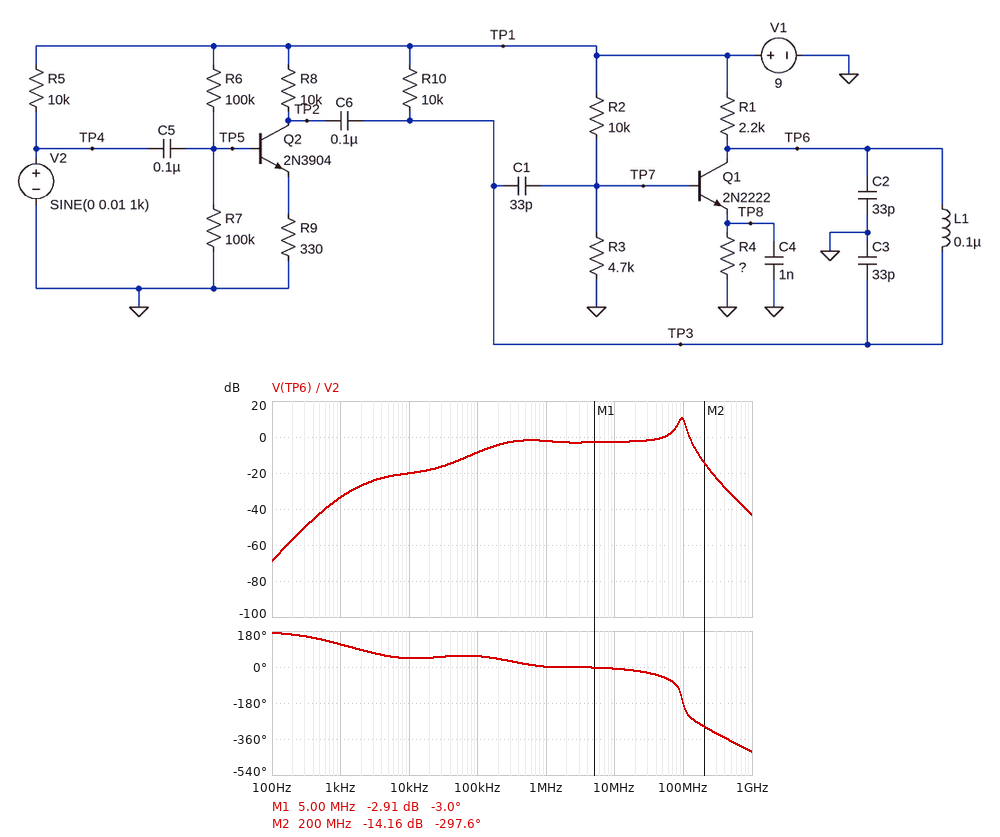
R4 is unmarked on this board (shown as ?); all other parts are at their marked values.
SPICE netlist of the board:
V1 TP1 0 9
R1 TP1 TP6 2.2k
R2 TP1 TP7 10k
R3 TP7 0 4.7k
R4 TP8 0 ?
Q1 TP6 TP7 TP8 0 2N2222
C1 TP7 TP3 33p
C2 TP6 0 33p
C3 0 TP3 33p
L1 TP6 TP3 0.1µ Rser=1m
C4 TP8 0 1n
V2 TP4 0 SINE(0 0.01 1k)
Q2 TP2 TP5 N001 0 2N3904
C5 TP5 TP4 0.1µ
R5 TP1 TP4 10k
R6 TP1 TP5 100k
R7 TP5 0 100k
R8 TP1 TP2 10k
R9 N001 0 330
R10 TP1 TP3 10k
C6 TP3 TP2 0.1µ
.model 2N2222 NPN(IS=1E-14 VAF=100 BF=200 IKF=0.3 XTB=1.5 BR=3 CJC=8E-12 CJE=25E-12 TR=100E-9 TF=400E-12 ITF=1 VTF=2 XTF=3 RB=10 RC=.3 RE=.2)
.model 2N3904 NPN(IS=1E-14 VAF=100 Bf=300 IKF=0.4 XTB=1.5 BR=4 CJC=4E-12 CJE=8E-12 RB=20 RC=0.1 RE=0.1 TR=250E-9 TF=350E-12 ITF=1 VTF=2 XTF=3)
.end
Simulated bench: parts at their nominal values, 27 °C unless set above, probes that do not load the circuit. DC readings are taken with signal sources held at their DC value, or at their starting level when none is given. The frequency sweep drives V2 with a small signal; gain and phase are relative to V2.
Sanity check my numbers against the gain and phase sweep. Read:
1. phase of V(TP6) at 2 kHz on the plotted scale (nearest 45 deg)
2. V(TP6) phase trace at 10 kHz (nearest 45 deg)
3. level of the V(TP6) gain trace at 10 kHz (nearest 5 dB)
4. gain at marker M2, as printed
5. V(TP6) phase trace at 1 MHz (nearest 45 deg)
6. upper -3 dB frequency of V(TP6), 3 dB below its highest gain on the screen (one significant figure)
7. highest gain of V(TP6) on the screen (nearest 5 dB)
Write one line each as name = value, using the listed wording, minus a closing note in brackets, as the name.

phase of V(TP6) at 2 kHz on the plotted scale = 90 deg
V(TP6) phase trace at 10 kHz = 45 deg
level of the V(TP6) gain trace at 10 kHz = -20 dB
gain at marker M2, as printed = -14.16 dB
V(TP6) phase trace at 1 MHz = 0 deg
upper -3 dB frequency of V(TP6), 3 dB below its highest gain on the screen = 100 MHz
highest gain of V(TP6) on the screen = 10 dB
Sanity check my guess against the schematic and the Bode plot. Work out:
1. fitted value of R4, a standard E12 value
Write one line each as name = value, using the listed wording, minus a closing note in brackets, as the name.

fitted value of R4, a standard E12 value = 2.2 kΩ
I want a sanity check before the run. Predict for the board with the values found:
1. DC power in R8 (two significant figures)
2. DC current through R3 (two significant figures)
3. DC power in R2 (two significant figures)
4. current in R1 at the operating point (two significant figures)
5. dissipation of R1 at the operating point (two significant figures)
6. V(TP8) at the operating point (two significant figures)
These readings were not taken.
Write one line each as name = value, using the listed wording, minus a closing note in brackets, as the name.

DC power in R8 = 7.5 mW
DC current through R3 = 610 µA
DC power in R2 = 3.8 mW
current in R1 at the operating point = 820 µA
dissipation of R1 at the operating point = 1.5 mW
V(TP8) at the operating point = 2.2 V
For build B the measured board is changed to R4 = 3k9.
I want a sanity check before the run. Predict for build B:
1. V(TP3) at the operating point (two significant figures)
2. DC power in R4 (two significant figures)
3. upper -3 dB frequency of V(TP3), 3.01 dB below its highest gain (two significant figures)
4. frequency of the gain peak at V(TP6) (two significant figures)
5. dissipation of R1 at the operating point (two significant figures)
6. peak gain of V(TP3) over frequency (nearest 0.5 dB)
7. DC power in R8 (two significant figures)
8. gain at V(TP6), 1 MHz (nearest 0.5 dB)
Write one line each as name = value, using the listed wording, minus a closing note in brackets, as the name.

V(TP3) at the operating point = 8.0 V
DC power in R4 = 1.3 mW
upper -3 dB frequency of V(TP3), 3.01 dB below its highest gain = 150 MHz
frequency of the gain peak at V(TP6) = 92 MHz
dissipation of R1 at the operating point = 480 µW
peak gain of V(TP3) over frequency = 1.0 dB
DC power in R8 = 7.5 mW
gain at V(TP6), 1 MHz = -2.5 dB
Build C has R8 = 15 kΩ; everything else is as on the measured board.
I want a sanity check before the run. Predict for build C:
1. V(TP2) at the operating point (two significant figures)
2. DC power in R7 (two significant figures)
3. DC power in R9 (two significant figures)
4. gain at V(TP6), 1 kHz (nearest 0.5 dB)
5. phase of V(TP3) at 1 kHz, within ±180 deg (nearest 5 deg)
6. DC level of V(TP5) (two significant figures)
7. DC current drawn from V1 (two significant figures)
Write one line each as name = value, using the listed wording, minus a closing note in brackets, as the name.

V(TP2) at the operating point = 250 mV
DC power in R7 = 7.6 µW
DC power in R9 = 140 µW
gain at V(TP6), 1 kHz = -28.0 dB
phase of V(TP3) at 1 kHz, within ±180 deg = 110 deg
DC level of V(TP5) = 870 mV
DC current drawn from V1 = 3.2 mA
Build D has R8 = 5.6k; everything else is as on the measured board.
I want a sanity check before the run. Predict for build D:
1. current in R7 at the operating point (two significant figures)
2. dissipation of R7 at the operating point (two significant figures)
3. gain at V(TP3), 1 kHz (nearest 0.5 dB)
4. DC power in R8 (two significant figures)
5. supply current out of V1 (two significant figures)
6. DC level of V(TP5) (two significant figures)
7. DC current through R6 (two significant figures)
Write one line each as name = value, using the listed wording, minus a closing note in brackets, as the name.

current in R7 at the operating point = 12 µA
dissipation of R7 at the operating point = 14 µW
gain at V(TP3), 1 kHz = -41.0 dB
DC power in R8 = 13 mW
supply current out of V1 = 4.1 mA
DC level of V(TP5) = 1.2 V
DC current through R6 = 78 µA
